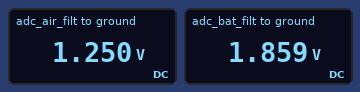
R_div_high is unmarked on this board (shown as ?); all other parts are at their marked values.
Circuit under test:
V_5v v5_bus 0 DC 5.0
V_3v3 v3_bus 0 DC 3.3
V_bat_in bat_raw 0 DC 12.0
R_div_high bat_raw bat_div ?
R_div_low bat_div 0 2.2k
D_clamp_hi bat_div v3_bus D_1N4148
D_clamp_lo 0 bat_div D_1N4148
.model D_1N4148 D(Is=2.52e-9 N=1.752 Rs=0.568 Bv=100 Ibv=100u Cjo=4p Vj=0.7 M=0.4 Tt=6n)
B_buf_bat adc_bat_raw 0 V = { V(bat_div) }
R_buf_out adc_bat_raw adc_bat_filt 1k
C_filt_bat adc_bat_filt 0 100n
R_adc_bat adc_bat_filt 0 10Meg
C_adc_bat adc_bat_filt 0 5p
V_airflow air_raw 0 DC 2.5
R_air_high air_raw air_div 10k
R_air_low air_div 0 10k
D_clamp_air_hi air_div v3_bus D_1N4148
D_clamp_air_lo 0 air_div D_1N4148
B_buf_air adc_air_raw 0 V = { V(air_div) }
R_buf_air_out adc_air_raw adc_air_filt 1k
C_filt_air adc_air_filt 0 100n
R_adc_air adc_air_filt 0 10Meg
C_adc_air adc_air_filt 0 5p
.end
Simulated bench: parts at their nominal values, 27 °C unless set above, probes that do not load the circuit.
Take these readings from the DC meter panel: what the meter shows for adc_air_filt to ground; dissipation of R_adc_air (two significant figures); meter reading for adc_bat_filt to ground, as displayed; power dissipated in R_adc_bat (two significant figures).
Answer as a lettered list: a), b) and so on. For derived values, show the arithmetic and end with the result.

a) 1.250 V
b) (1.25 V)^2 / 10 MΩ = 160 nW
c) 1.859 V
d) (1.859 V)^2 / 10 MΩ = 350 nW
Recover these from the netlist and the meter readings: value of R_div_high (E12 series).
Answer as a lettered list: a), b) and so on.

a) 12 kΩ
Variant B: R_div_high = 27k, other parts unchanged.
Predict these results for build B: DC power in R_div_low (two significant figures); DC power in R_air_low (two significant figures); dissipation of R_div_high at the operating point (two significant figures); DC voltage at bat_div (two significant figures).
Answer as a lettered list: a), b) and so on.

a) 370 µW
b) 160 µW
c) 4.6 mW
d) 900 mV
